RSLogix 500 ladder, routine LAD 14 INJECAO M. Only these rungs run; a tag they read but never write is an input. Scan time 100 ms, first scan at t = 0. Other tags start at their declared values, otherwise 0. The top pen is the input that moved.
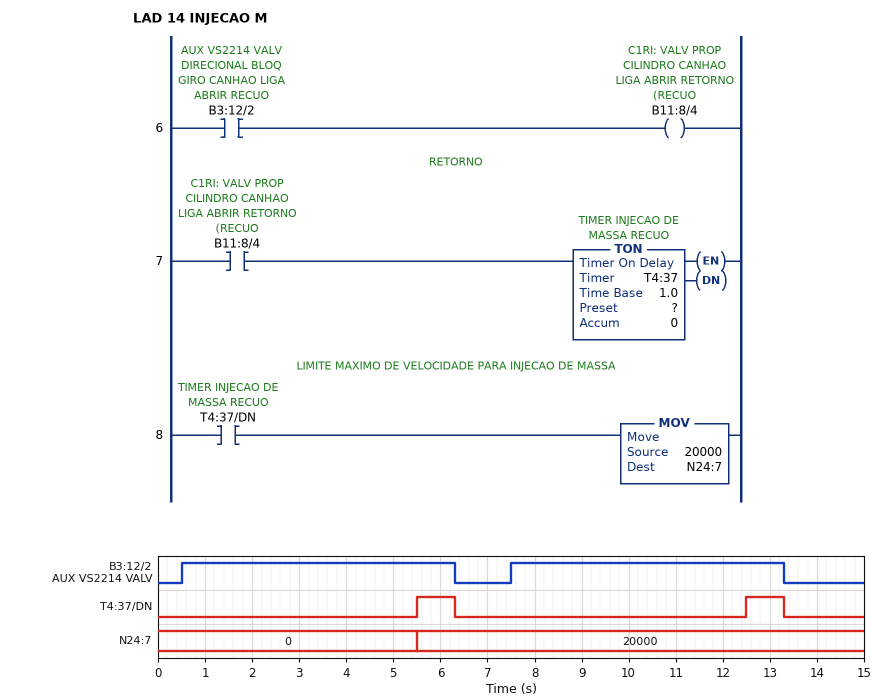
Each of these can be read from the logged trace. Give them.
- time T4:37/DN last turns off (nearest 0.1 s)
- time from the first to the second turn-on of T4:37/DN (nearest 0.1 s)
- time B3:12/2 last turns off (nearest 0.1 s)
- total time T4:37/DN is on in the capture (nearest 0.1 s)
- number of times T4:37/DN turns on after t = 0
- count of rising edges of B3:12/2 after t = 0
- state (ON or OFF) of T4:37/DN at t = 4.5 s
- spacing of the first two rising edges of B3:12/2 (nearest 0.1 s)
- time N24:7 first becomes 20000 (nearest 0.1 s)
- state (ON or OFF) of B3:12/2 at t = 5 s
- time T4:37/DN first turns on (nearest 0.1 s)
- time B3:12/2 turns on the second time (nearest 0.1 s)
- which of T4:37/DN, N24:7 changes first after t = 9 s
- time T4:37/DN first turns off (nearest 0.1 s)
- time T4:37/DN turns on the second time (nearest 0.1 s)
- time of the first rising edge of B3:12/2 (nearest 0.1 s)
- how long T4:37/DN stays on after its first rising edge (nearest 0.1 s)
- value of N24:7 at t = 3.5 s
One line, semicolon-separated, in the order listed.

13.3 s; 7.0 s; 13.3 s; 1.6 s; 2; 2; OFF; 7.0 s; 5.5 s; ON; 5.5 s; 7.5 s; T4:37/DN; 6.3 s; 12.5 s; 0.5 s; 0.8 s; 0
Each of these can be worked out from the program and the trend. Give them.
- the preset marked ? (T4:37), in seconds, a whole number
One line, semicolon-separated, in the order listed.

5 s
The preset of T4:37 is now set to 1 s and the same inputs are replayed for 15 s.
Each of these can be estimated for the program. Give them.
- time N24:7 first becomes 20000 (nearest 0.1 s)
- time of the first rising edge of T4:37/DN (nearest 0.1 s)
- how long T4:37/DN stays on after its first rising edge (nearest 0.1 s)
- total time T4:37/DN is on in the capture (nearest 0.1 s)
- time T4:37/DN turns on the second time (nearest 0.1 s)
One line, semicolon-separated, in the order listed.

1.5 s; 1.5 s; 4.8 s; 9.6 s; 8.5 s
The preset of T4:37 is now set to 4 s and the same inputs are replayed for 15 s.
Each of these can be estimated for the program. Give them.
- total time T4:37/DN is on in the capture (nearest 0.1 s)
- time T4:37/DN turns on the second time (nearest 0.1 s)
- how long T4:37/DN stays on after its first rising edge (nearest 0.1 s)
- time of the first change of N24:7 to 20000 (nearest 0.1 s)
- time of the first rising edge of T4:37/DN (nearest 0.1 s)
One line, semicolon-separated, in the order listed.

3.6 s; 11.5 s; 1.8 s; 4.5 s; 4.5 s
